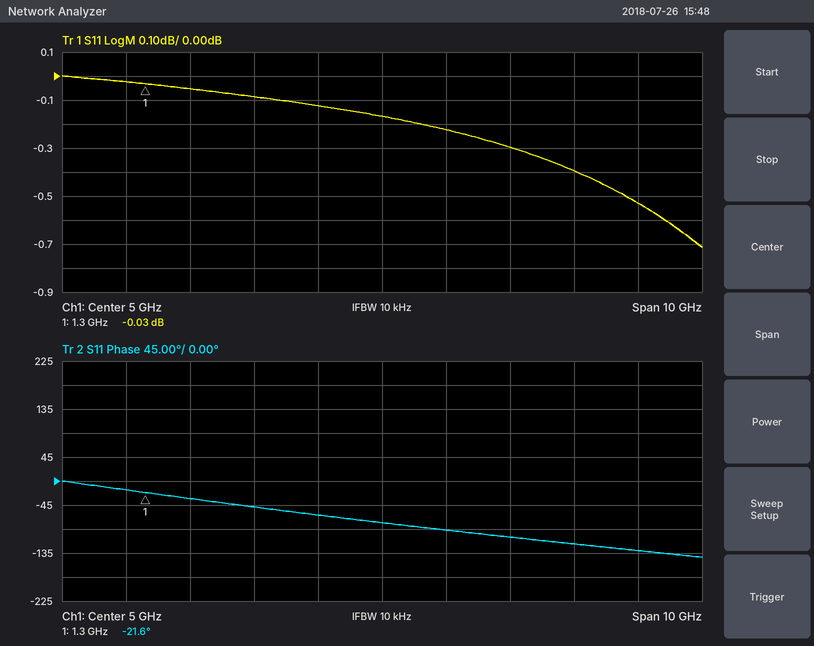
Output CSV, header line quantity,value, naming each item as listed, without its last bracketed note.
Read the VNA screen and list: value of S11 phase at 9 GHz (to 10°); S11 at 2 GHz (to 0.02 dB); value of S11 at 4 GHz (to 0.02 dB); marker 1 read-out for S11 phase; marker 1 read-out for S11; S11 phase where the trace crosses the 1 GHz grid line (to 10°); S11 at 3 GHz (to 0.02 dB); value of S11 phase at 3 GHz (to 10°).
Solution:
quantity,value
value of S11 phase at 9 GHz,-130°
S11 at 2 GHz,-0.06 dB
value of S11 at 4 GHz,-0.12 dB
marker 1 read-out for S11 phase,-21.6°
marker 1 read-out for S11,-0.03 dB
S11 phase where the trace crosses the 1 GHz grid line,-20°
S11 at 3 GHz,-0.08 dB
value of S11 phase at 3 GHz,-50°
